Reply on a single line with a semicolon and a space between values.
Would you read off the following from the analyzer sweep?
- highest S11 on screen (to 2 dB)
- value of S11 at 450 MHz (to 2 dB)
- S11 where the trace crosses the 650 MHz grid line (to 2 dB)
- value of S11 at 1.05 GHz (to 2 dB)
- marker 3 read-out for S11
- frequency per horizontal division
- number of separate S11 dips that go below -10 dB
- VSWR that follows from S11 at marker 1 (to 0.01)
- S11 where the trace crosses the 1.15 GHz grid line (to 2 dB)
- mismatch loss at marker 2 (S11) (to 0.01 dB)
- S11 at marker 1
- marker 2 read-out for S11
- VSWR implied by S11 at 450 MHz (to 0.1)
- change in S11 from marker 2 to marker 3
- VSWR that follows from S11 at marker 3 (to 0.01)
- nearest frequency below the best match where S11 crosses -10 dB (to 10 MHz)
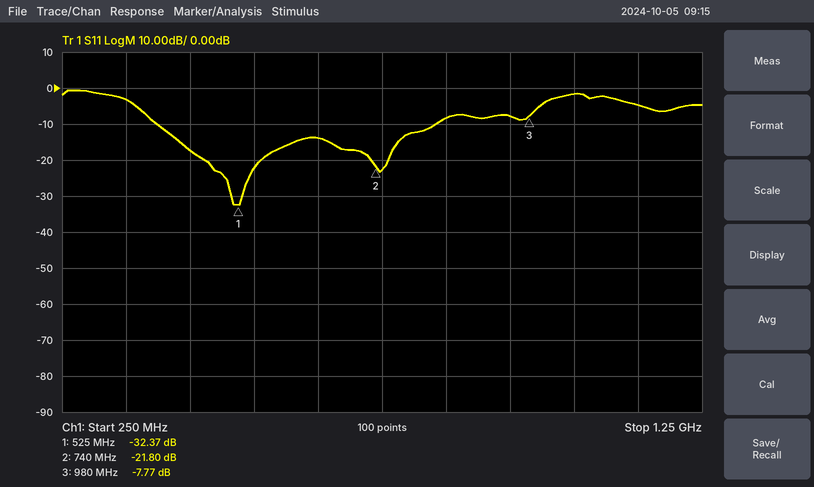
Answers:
0 dB; -18 dB; -14 dB; -2 dB; -7.77 dB; 100 MHz; 2; 1.05; -4 dB; 0.03 dB; -32.37 dB; -21.80 dB; 1.3; 14.03 dB; 2.38; 400 MHz
